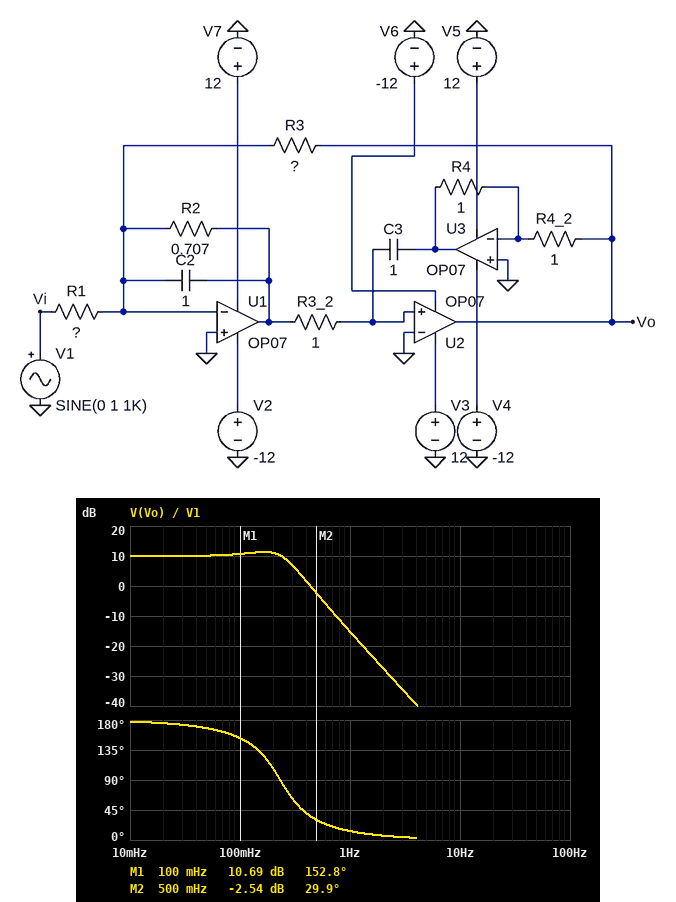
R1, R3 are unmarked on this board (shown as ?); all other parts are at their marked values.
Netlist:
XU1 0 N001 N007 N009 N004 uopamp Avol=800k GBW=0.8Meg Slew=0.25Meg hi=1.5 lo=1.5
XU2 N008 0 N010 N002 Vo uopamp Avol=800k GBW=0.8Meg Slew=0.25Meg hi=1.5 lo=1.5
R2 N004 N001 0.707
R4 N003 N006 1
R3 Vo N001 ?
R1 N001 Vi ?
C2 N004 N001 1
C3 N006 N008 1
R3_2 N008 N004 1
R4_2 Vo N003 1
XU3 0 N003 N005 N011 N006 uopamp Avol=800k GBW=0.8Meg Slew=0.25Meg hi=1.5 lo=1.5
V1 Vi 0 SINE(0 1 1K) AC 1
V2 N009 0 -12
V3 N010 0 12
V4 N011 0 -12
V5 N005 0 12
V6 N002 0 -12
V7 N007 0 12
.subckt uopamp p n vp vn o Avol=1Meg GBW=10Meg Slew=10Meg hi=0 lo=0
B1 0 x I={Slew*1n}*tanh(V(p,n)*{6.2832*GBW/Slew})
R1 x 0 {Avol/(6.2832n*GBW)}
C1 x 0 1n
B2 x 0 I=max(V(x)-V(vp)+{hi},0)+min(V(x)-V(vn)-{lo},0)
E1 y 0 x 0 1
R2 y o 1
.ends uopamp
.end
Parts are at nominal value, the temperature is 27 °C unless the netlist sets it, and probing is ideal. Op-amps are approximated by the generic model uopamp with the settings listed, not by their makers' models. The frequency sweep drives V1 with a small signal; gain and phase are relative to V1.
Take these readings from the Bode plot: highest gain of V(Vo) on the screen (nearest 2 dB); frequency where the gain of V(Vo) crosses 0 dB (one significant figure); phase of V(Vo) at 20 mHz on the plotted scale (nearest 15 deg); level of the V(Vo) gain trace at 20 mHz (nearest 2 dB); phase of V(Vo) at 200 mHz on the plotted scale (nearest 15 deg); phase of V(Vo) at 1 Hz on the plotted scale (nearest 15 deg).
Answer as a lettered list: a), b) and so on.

a) 12 dB
b) 400 mHz
c) 180 deg
d) 10 dB
e) 105 deg
f) 15 deg
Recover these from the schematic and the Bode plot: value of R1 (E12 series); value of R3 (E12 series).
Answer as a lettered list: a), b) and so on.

a) 0.15 Ω
b) 0.47 Ω
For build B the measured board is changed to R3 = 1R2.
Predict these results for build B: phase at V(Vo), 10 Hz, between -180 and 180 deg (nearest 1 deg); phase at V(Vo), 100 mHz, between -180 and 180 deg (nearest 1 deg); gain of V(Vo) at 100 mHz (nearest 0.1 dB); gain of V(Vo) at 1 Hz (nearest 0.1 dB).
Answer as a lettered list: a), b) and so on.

a) 1 deg
b) 116 deg
c) 16.6 dB
d) -15.5 dB
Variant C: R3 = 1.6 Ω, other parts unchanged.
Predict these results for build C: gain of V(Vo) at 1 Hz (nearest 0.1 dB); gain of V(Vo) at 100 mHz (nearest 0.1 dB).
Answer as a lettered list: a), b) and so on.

a) -15.5 dB
b) 17.2 dB
